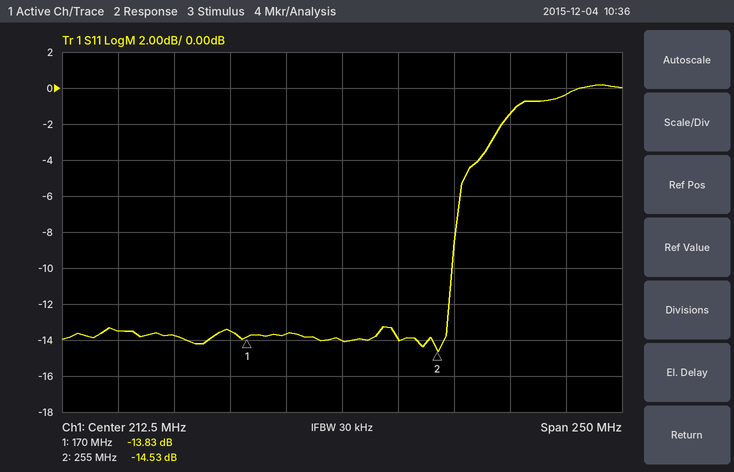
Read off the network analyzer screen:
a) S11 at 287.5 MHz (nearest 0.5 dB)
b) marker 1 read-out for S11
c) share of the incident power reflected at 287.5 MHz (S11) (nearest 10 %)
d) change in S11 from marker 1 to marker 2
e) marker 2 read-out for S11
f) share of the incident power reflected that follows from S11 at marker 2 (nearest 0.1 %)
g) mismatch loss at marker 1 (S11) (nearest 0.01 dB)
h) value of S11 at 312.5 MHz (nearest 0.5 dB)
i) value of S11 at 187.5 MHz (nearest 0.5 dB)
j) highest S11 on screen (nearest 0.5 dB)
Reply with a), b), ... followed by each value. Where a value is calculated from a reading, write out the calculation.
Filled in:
a) -1.5 dB
b) -13.83 dB
c) 10^(-1.5/10) ≈ 70.8 %, so 70 % to the nearest 10 %
d) -14.53 − (-13.83) = -0.70 dB
e) -14.53 dB
f) 10^(-14.53/10) ≈ 3.5 %
g) −10 log10(1 − 10^(-13.83/10)) ≈ 0.18 dB
h) -0.5 dB
i) -13.5 dB
j) 0.0 dB
